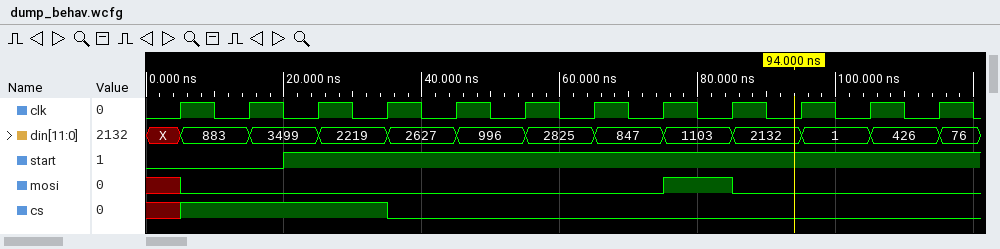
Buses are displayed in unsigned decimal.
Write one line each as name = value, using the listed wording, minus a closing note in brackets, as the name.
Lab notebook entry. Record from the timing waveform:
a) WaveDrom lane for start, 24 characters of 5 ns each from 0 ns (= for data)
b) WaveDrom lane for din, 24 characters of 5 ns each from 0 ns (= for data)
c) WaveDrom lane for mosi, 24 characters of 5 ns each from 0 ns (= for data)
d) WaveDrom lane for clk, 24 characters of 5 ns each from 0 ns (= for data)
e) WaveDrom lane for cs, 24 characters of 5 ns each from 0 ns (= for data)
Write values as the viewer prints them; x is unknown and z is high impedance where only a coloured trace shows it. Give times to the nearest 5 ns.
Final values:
WaveDrom lane for start, 24 characters of 5 ns each from 0 ns = {name: 'start', wave: '0...1...................'}
WaveDrom lane for din, 24 characters of 5 ns each from 0 ns = {name: 'din', wave: 'x=.=.=.=.=.=.=.=.=.=.=.=', data: '883 3499 2219 2627 996 2825 847 1103 2132 1 426 76'}
WaveDrom lane for mosi, 24 characters of 5 ns each from 0 ns = {name: 'mosi', wave: 'x0.............1.0......'}
WaveDrom lane for clk, 24 characters of 5 ns each from 0 ns = {name: 'clk', wave: '010101010101010101010101'}
WaveDrom lane for cs, 24 characters of 5 ns each from 0 ns = {name: 'cs', wave: 'x1.....0................'}
